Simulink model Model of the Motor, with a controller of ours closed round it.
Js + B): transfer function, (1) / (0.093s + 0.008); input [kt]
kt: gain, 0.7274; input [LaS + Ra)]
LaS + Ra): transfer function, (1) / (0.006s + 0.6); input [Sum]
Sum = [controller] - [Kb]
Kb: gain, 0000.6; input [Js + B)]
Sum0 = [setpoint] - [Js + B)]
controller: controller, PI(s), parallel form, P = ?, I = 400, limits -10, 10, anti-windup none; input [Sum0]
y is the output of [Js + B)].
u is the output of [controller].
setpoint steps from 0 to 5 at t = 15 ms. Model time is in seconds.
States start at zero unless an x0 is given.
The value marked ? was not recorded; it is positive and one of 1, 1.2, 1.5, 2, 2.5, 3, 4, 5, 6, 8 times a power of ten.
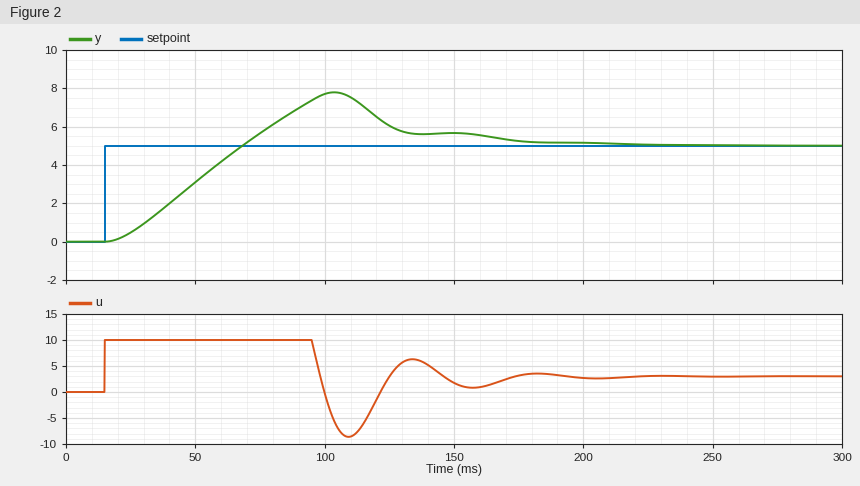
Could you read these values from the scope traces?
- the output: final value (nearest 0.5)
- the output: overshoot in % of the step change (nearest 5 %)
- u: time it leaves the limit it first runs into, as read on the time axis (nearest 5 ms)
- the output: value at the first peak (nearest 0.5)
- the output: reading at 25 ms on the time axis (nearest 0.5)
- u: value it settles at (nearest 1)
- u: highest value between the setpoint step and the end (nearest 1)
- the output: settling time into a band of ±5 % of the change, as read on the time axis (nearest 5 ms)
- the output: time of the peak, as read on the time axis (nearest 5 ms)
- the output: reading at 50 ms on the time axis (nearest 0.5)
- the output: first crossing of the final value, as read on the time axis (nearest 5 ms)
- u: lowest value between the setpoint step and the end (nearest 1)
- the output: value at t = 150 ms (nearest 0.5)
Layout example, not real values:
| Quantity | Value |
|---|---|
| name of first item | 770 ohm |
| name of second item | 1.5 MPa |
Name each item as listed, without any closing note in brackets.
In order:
| Quantity | Value |
|---|---|
| the output: final value | 5.0 |
| the output: overshoot in % of the step change | 55 % |
| u: time it leaves the limit it first runs into, as read on the time axis | 95 ms |
| the output: value at the first peak | 8.0 |
| the output: reading at 25 ms on the time axis | 0.5 |
| u: value it settles at | 3 |
| u: highest value between the setpoint step and the end | 10 |
| the output: settling time into a band of ±5 % of the change, as read on the time axis | 175 ms |
| the output: time of the peak, as read on the time axis | 105 ms |
| the output: reading at 50 ms on the time axis | 3.0 |
| the output: first crossing of the final value, as read on the time axis | 70 ms |
| u: lowest value between the setpoint step and the end | -9 |
| the output: value at t = 150 ms | 5.5 |
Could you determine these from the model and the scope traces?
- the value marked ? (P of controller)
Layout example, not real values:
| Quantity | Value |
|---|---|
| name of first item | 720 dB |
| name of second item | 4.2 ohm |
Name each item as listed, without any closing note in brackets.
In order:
| Quantity | Value |
|---|---|
| the value marked ? | 15 |
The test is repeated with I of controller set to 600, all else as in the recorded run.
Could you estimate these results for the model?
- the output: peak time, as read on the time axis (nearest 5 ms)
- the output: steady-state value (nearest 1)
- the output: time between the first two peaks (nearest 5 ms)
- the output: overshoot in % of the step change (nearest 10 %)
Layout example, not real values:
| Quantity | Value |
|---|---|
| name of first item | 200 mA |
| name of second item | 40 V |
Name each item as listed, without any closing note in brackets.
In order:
| Quantity | Value |
|---|---|
| the output: peak time, as read on the time axis | 110 ms |
| the output: steady-state value | 5 |
| the output: time between the first two peaks | 55 ms |
| the output: overshoot in % of the step change | 70 % |
